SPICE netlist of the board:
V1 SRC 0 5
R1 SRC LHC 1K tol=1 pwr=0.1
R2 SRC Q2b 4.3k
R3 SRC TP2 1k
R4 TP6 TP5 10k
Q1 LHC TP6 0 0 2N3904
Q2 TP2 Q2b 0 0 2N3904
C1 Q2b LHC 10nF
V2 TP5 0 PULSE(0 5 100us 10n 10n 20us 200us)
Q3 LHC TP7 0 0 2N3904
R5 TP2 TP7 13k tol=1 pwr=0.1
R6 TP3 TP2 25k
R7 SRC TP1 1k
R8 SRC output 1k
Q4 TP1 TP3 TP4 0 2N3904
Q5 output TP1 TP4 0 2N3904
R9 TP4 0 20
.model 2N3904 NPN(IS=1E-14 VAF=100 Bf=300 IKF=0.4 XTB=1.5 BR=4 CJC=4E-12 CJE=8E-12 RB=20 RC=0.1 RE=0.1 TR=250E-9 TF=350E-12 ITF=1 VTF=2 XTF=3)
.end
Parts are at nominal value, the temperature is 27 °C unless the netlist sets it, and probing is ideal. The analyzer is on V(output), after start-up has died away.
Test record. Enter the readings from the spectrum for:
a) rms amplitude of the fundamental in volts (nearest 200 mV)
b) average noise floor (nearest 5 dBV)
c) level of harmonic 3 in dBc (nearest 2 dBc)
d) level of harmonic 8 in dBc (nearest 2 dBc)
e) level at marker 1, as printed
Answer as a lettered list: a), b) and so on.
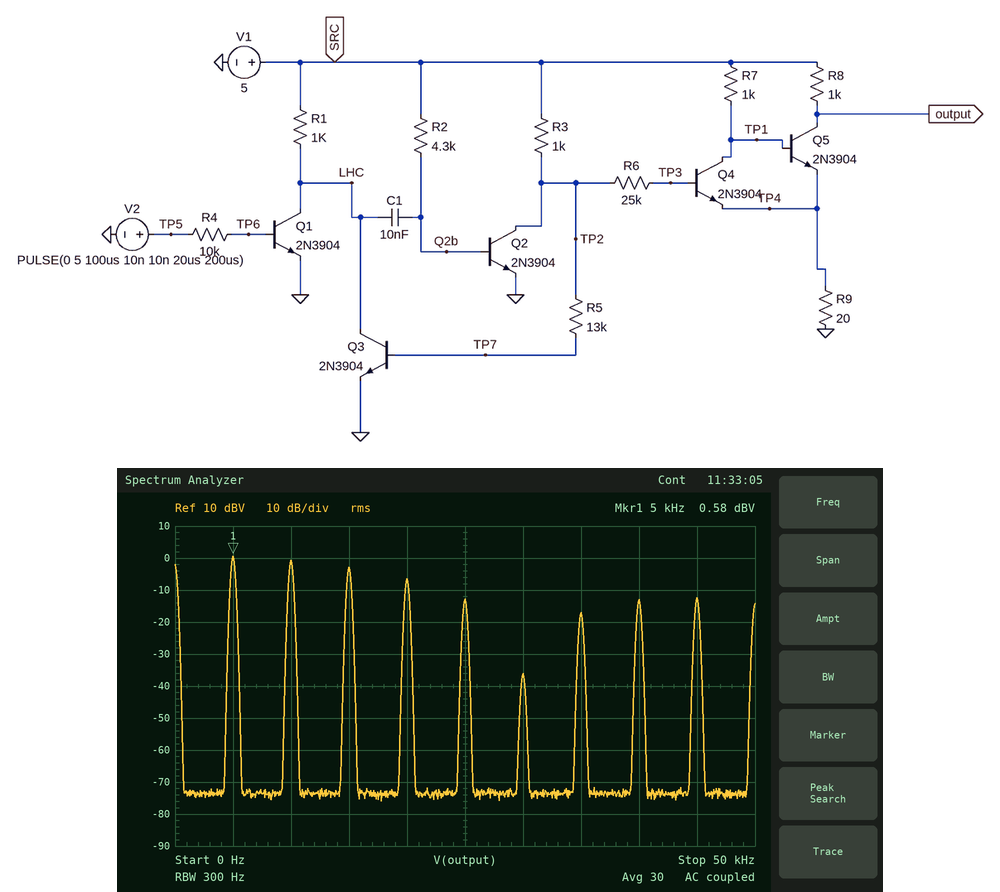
a) 1.0 V
b) -75 dBV
c) -4 dBc
d) -14 dBc
e) 0.58 dBV
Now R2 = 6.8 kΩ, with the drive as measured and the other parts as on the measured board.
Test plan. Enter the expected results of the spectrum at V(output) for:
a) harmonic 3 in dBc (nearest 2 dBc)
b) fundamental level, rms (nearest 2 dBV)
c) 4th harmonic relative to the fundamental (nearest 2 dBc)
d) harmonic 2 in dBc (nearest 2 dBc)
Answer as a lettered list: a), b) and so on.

a) -10 dBc
b) 4 dBV
c) -28 dBc
d) -4 dBc
